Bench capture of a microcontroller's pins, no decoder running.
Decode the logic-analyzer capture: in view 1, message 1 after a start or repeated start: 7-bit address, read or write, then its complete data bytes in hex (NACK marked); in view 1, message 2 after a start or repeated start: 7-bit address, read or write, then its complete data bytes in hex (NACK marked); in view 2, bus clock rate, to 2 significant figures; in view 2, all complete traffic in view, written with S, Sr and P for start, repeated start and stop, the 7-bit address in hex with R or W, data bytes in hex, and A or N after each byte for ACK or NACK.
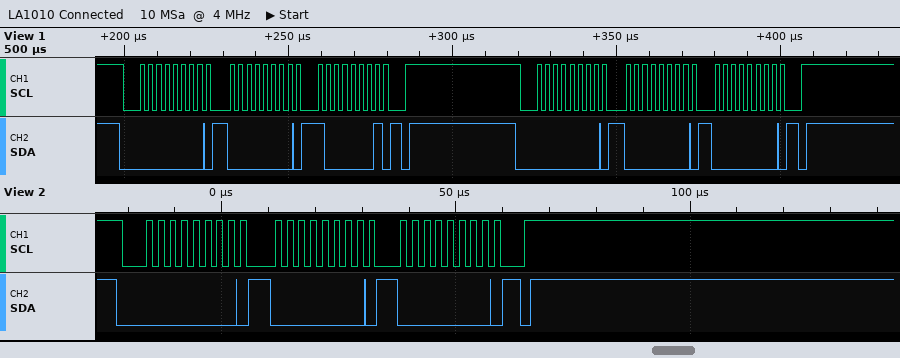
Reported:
0x00 write: 00 81
0x00 write: 00 00
400 kHz
S 00W A 00 A 00 A P
